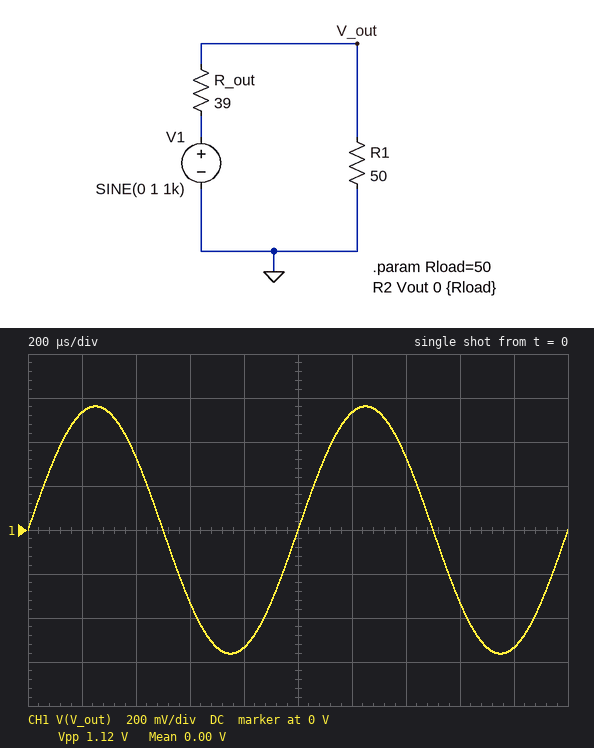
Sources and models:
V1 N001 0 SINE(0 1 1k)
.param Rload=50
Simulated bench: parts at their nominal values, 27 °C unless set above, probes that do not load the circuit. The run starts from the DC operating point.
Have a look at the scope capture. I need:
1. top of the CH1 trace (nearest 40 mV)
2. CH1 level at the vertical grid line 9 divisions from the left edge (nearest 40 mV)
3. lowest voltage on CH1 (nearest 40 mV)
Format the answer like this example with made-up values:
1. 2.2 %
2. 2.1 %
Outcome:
1. 560 mV
2. -520 mV
3. -560 mV
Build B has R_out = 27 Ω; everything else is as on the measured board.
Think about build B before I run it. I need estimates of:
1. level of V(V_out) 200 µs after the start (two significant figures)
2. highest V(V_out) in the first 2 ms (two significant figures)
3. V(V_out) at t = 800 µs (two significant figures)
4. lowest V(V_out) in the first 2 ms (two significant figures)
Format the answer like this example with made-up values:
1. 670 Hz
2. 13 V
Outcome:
1. 620 mV
2. 650 mV
3. -620 mV
4. -650 mV
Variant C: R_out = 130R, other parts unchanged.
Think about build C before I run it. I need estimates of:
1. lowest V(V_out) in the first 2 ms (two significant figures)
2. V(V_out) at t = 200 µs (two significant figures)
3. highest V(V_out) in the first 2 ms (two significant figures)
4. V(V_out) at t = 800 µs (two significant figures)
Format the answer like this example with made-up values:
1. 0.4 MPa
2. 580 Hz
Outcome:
1. -280 mV
2. 260 mV
3. 280 mV
4. -260 mV
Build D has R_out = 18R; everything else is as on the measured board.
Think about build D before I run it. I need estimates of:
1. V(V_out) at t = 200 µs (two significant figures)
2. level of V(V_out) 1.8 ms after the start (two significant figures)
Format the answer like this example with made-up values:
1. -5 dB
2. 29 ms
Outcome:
1. 700 mV
2. -700 mV
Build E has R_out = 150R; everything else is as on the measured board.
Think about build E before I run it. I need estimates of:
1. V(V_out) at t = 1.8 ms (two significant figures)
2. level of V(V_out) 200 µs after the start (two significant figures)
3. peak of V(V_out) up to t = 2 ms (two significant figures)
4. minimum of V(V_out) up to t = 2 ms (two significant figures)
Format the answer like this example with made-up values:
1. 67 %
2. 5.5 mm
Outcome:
1. -240 mV
2. 240 mV
3. 250 mV
4. -250 mV
